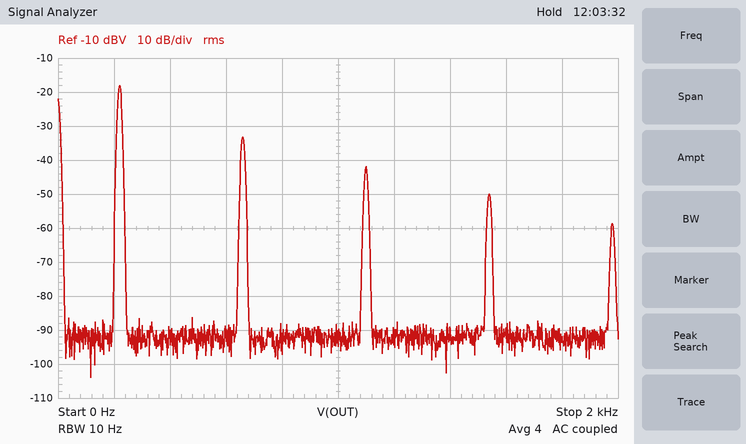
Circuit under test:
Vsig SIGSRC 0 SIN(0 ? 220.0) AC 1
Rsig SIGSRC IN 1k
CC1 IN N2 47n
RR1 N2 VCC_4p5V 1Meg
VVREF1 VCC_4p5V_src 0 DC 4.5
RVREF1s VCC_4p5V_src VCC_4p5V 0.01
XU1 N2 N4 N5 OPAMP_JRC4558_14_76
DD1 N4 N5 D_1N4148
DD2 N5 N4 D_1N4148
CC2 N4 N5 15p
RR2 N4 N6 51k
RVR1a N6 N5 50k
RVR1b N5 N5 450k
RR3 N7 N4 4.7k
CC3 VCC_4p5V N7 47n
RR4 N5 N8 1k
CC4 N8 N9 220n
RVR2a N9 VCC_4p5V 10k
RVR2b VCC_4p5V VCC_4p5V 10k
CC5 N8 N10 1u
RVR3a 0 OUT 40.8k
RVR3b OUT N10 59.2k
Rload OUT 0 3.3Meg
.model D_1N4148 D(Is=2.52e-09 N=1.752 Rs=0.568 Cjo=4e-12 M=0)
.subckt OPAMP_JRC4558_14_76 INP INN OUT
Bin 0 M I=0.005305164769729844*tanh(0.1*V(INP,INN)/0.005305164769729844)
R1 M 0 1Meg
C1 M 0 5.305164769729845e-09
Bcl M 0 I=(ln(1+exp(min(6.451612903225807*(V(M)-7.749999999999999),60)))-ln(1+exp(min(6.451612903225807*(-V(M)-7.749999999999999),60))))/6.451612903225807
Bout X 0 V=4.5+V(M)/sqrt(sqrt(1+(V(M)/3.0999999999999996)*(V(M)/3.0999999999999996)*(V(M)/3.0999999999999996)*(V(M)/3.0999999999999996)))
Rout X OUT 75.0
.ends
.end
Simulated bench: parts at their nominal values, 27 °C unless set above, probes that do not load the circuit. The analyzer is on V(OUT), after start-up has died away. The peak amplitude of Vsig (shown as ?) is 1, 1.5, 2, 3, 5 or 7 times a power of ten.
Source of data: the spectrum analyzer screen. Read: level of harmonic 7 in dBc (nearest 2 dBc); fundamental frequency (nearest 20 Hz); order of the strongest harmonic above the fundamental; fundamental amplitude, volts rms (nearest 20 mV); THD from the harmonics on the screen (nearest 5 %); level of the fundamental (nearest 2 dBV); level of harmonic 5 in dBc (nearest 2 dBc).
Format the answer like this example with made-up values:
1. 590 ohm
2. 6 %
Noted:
1. -32 dBc
2. 220 Hz
3. 3
4. 120 mV
5. 20 %
6. -18 dBV
7. -24 dBc
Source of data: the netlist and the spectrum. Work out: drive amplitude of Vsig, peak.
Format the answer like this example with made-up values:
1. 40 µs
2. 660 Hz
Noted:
1. 150 mV
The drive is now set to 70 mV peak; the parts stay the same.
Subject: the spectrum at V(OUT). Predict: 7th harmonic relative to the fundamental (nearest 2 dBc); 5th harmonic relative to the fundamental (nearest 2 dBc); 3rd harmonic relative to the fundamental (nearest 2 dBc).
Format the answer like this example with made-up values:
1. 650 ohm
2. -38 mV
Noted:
1. -54 dBc
2. -38 dBc
3. -20 dBc
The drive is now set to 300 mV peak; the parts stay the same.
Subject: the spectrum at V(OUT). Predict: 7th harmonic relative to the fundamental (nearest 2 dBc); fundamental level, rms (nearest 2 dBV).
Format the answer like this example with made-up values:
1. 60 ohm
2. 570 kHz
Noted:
1. -26 dBc
2. -16 dBV
